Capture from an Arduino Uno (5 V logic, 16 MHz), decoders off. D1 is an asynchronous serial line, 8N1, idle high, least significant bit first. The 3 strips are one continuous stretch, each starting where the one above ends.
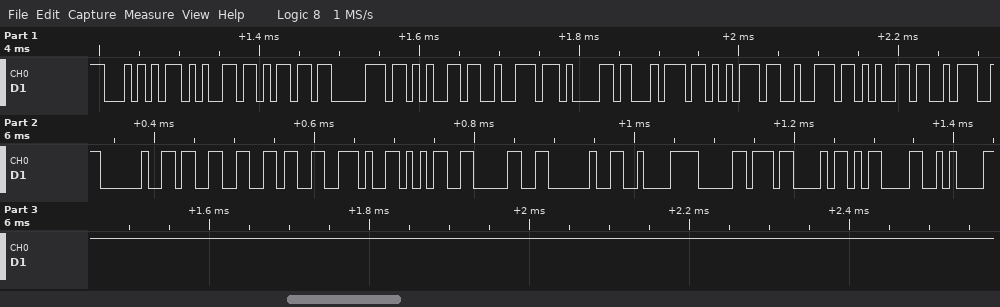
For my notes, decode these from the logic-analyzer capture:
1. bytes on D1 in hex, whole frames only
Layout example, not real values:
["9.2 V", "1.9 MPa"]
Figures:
["0x54 0x65 0x6D 0x70 0x65 0x72 0x61 0x74 0x75 0x72 0x65 0x3A 0x20 0x33 0x36 0x2E 0x35 0x30 0x20 0xC2 0xB0 0x43 0x0D 0x0A"]
